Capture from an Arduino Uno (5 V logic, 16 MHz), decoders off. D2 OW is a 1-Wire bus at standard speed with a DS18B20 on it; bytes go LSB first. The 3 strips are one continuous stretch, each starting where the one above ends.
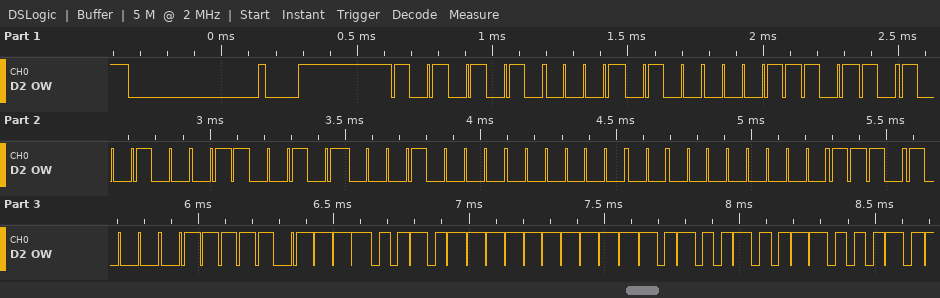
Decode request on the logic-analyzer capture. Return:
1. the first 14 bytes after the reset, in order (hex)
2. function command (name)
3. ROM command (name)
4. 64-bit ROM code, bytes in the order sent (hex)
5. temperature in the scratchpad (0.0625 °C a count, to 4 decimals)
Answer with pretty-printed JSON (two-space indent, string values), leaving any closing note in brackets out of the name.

{
  "the first 14 bytes after the reset, in order": "55 28 B8 25 A6 08 00 00 17 BE A7 FF 4B 46",
  "function command": "Read Scratchpad",
  "ROM command": "Match ROM",
  "64-bit ROM code, bytes in the order sent": "28 B8 25 A6 08 00 00 17",
  "temperature in the scratchpad": "-5.5625 °C"
}
